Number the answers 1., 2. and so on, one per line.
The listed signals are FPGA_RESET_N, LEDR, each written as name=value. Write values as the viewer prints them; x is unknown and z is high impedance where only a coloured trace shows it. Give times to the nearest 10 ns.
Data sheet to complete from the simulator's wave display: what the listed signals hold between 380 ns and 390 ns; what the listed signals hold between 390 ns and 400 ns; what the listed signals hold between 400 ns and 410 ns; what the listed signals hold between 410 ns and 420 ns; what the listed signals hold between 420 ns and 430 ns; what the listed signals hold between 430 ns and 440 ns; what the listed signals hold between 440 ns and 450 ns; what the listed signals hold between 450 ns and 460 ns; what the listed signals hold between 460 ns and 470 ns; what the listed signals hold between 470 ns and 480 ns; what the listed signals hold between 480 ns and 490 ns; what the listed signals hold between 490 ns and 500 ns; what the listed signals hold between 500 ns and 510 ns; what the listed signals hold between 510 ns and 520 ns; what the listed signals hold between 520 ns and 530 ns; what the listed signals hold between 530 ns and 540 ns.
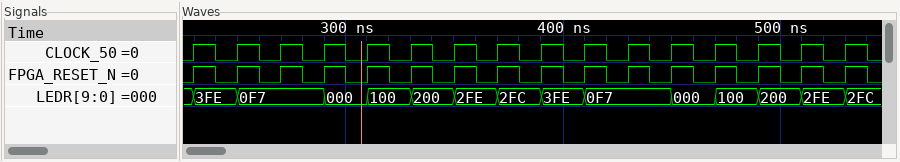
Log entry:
1. FPGA_RESET_N=0, LEDR=2FC
2. FPGA_RESET_N=1, LEDR=3FE
3. FPGA_RESET_N=0, LEDR=3FE
4. FPGA_RESET_N=1, LEDR=0F7
5. FPGA_RESET_N=0, LEDR=0F7
6. FPGA_RESET_N=1, LEDR=0F7
7. FPGA_RESET_N=0, LEDR=0F7
8. FPGA_RESET_N=1, LEDR=000
9. FPGA_RESET_N=0, LEDR=000
10. FPGA_RESET_N=1, LEDR=100
11. FPGA_RESET_N=0, LEDR=100
12. FPGA_RESET_N=1, LEDR=200
13. FPGA_RESET_N=0, LEDR=200
14. FPGA_RESET_N=1, LEDR=2FE
15. FPGA_RESET_N=0, LEDR=2FE
16. FPGA_RESET_N=1, LEDR=2FC
